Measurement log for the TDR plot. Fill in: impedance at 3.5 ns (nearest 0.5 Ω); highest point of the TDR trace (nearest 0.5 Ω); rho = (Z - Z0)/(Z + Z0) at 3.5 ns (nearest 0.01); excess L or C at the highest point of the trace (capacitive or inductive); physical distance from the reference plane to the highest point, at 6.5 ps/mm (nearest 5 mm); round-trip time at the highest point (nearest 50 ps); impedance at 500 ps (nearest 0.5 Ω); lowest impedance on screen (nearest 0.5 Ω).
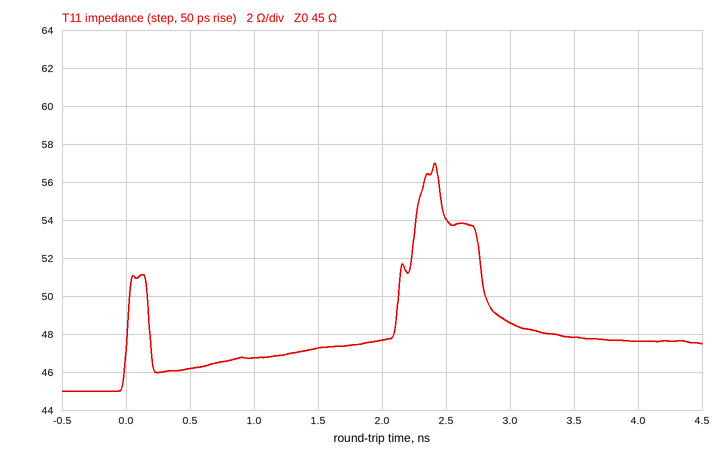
48.0 Ω
57.0 Ω
+0.03
inductive
185 mm
2.40 ns
46.0 Ω
45.0 Ω
